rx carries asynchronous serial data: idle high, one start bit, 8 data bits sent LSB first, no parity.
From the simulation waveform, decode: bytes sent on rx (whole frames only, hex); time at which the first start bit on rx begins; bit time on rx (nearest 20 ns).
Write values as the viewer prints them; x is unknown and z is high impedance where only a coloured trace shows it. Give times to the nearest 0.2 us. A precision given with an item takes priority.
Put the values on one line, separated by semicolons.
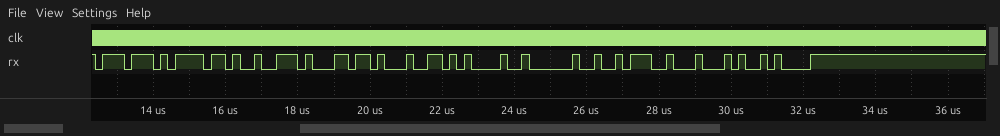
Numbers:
77, 6F, 72, 6C, 64, 21, 20, 3A, 44, 0A; 12.4 us; 200 ns
